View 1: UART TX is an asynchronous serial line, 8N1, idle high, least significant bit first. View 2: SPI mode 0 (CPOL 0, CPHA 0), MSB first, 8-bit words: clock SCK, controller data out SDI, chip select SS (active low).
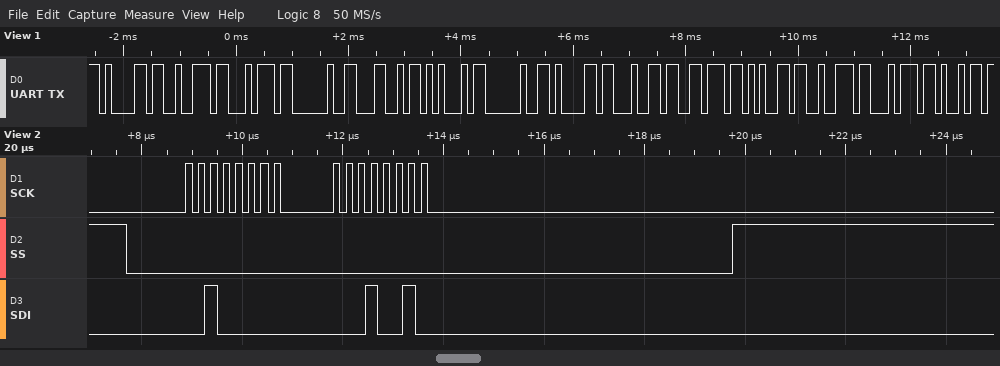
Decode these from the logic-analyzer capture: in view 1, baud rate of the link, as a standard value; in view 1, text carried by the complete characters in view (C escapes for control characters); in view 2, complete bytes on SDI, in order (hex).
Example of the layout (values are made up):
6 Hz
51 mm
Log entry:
9600 baud
"art LE adverti"
20 12
